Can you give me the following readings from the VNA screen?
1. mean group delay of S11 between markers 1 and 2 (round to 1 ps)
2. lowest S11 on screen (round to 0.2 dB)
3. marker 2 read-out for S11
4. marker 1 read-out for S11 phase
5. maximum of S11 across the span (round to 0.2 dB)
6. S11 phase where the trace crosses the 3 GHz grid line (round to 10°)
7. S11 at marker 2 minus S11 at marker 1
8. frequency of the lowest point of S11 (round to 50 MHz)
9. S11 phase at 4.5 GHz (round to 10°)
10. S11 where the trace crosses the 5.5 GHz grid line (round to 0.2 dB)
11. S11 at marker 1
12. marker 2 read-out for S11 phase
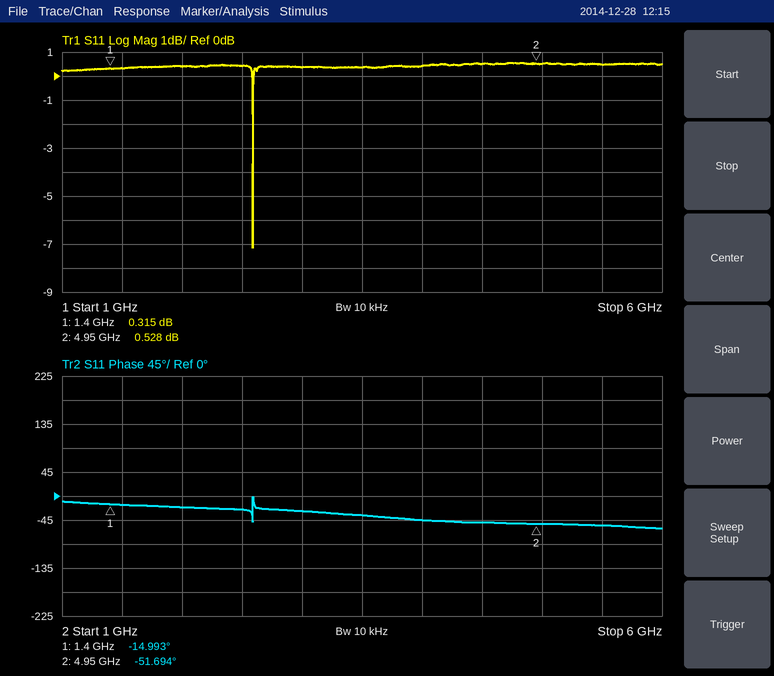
29 ps
-7.2 dB
0.528 dB
-14.993°
0.6 dB
-30°
0.213 dB
2.60 GHz
-50°
0.4 dB
0.315 dB
-51.694°
